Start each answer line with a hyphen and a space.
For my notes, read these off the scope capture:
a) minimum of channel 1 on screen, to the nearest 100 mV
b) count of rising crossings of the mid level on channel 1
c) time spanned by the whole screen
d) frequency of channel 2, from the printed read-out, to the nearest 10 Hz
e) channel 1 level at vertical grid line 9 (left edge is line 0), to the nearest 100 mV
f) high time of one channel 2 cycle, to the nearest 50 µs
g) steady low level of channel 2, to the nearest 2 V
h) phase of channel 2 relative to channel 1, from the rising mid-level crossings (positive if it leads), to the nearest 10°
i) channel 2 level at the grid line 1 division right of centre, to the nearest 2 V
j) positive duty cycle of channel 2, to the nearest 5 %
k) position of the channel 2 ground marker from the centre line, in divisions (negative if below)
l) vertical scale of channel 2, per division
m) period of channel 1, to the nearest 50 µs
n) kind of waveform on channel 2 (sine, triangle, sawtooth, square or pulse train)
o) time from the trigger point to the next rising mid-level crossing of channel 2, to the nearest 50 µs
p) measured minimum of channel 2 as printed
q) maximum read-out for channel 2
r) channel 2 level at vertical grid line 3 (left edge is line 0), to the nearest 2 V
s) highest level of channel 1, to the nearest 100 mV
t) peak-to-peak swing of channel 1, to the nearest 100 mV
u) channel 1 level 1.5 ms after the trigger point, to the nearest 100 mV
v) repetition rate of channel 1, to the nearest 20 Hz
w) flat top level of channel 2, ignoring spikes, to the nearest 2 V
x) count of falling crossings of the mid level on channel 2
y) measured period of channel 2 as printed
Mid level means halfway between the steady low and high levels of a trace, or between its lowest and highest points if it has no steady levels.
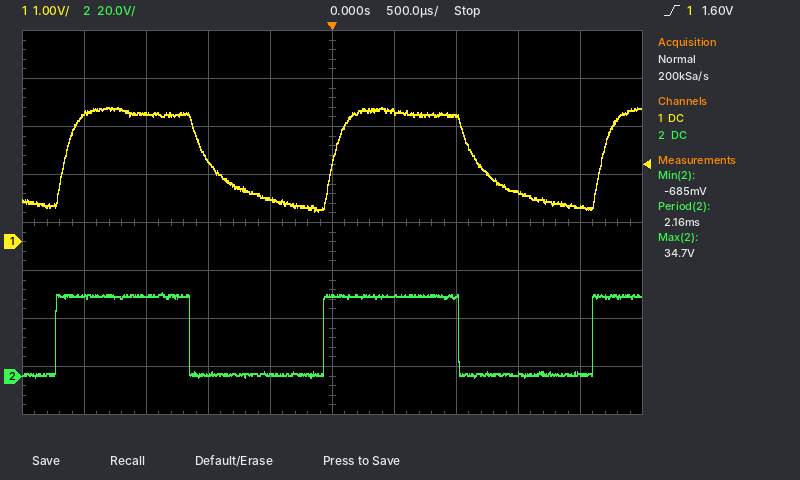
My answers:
- 600 mV
- 3
- 5 ms
- 460 Hz
- 700 mV
- 1.10 ms
- 0 V
- +10°
- 34 V
- 50 %
- -3.2 div
- 20 V
- 2.15 ms
- square
- 2.10 ms
- -685 mV
- 34.7 V
- 0 V
- 2.8 V
- 2.2 V
- 1.0 V
- 460 Hz
- 34 V
- 2
- 2.16 ms
